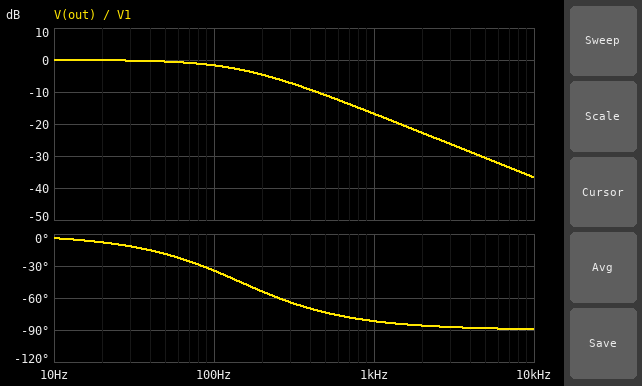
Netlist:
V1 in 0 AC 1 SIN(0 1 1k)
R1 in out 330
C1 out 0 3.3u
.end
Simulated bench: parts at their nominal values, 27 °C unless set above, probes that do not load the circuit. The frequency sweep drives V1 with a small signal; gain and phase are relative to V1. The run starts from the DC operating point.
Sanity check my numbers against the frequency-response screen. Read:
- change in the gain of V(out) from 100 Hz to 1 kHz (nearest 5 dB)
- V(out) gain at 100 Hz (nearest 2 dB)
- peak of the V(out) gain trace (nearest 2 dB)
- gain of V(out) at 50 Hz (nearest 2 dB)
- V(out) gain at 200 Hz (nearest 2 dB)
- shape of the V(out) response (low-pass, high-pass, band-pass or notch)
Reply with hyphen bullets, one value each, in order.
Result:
- -15 dB
- -2 dB
- 0 dB
- 0 dB
- -4 dB
- low-pass
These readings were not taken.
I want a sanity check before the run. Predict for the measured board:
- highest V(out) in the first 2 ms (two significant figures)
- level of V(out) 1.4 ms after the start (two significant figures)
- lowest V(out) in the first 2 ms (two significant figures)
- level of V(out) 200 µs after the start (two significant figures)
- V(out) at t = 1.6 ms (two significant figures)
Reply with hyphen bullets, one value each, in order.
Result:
- 240 mV
- 170 mV
- -120 mV
- 95 mV
- 140 mV
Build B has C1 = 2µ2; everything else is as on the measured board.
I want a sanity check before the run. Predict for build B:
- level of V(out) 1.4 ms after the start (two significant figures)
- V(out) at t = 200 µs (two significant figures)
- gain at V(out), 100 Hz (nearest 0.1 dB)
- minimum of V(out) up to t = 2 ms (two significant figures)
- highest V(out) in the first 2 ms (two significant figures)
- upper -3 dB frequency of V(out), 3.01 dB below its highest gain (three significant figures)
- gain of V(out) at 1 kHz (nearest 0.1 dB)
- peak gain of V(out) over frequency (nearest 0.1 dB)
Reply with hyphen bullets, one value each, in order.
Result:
- 230 mV
- 140 mV
- -0.8 dB
- -200 mV
- 330 mV
- 219 Hz
- -13.4 dB
- 0 dB
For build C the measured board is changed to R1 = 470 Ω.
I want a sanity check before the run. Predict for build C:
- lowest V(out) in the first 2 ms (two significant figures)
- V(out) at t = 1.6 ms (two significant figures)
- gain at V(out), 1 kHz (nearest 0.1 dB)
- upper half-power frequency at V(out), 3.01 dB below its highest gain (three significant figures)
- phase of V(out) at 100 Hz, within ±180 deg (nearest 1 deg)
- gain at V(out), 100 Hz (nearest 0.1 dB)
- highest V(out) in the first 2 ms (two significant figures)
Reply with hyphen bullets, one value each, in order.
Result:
- -74 mV
- 110 mV
- -19.8 dB
- 103 Hz
- -44 deg
- -2.9 dB
- 180 mV
